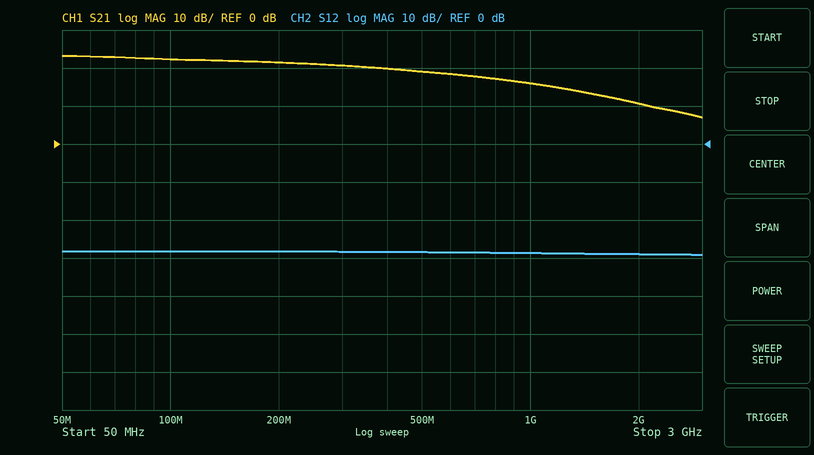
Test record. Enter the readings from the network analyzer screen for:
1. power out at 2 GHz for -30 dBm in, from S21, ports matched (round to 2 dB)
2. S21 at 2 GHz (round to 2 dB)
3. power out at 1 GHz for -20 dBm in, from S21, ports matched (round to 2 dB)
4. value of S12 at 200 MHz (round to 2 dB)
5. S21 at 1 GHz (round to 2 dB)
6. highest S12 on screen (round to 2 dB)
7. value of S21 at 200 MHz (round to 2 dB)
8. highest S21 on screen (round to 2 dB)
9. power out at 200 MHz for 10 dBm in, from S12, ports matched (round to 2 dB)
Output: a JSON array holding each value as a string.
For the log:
["-20 dBm", "10 dB", "-4 dBm", "-28 dB", "16 dB", "-28 dB", "22 dB", "24 dB", "-18 dBm"]
